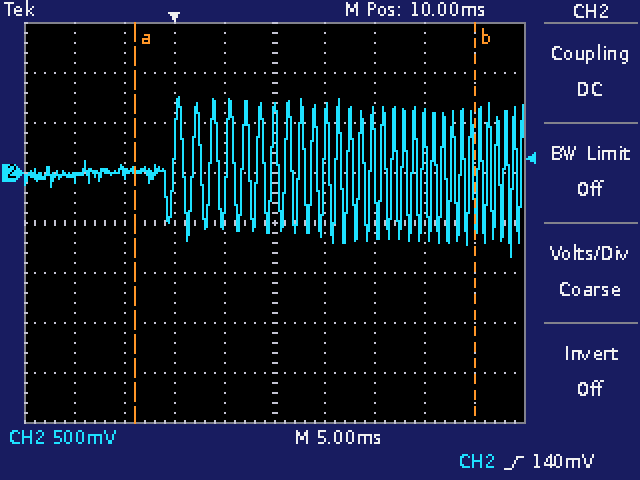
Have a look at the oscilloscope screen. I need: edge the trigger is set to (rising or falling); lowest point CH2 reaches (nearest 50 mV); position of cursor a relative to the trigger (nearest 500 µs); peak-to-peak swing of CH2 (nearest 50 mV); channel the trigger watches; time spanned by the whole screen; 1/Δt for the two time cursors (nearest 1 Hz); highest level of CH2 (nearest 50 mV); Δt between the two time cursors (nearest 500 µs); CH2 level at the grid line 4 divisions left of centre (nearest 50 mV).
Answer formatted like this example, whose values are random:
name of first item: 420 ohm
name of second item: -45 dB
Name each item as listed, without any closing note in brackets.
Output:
edge the trigger is set to: rising
lowest point CH2 reaches: -850 mV
position of cursor a relative to the trigger: -4.0 ms
peak-to-peak swing of CH2: 1.60 V
channel the trigger watches: CH2
time spanned by the whole screen: 50 ms
1/Δt for the two time cursors: 29 Hz
highest level of CH2: 750 mV
Δt between the two time cursors: 34.0 ms
CH2 level at the grid line 4 divisions left of centre: -50 mV
